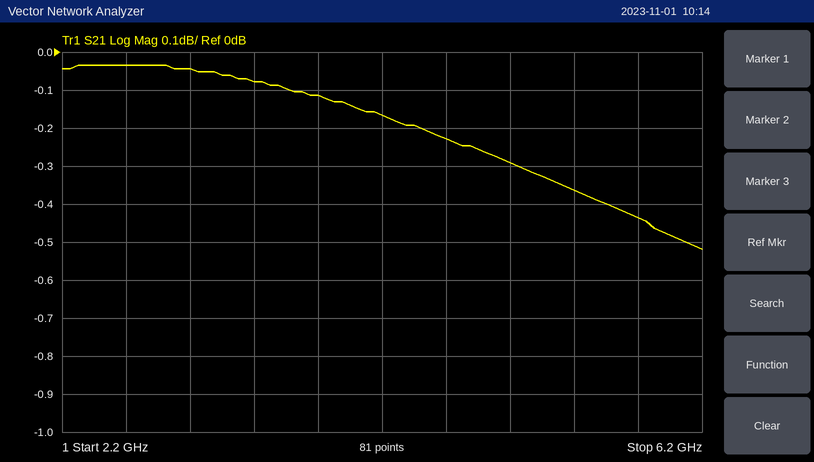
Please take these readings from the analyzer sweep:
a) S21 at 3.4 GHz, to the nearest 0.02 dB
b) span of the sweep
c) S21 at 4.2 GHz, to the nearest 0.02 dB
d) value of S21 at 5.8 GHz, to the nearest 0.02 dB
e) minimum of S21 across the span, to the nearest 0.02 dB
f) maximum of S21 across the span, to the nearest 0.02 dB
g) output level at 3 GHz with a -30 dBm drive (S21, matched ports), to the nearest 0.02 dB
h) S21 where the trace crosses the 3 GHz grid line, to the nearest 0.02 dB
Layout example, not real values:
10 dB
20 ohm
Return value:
-0.08 dB
4 GHz
-0.16 dB
-0.44 dB
-0.52 dB
-0.04 dB
-30.04 dBm
-0.04 dB
